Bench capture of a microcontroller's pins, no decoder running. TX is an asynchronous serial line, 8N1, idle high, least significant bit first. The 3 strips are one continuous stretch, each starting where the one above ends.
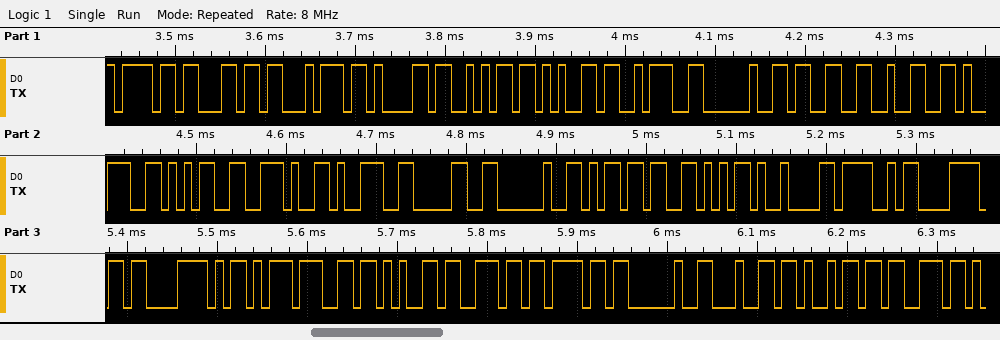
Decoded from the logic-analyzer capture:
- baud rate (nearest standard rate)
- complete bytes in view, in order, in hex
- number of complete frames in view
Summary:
115200 baud
6F 6C 74 61 6A 65 3A 20 33 32 39 35 2E 39 30 20 6D 56 09 4F 78 C3 AD 67 65 6E 6F 20 64 69 73
31
